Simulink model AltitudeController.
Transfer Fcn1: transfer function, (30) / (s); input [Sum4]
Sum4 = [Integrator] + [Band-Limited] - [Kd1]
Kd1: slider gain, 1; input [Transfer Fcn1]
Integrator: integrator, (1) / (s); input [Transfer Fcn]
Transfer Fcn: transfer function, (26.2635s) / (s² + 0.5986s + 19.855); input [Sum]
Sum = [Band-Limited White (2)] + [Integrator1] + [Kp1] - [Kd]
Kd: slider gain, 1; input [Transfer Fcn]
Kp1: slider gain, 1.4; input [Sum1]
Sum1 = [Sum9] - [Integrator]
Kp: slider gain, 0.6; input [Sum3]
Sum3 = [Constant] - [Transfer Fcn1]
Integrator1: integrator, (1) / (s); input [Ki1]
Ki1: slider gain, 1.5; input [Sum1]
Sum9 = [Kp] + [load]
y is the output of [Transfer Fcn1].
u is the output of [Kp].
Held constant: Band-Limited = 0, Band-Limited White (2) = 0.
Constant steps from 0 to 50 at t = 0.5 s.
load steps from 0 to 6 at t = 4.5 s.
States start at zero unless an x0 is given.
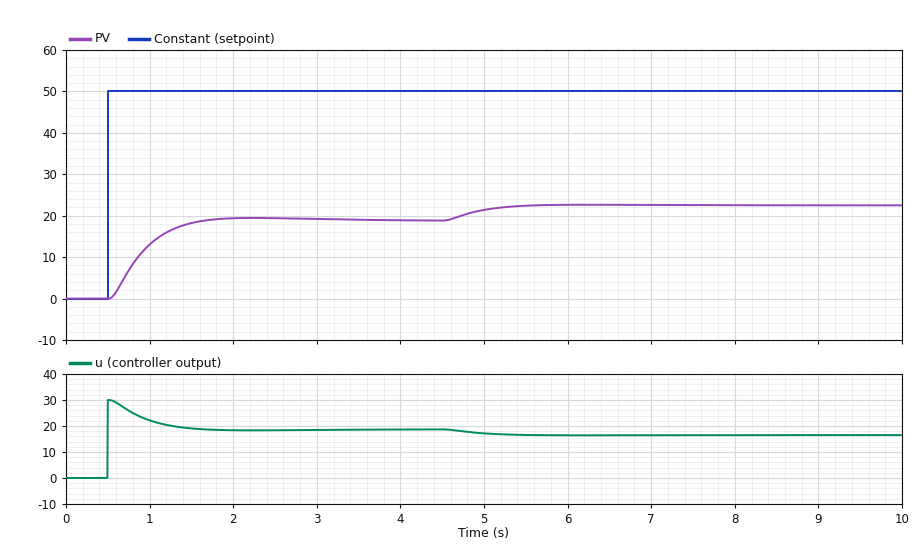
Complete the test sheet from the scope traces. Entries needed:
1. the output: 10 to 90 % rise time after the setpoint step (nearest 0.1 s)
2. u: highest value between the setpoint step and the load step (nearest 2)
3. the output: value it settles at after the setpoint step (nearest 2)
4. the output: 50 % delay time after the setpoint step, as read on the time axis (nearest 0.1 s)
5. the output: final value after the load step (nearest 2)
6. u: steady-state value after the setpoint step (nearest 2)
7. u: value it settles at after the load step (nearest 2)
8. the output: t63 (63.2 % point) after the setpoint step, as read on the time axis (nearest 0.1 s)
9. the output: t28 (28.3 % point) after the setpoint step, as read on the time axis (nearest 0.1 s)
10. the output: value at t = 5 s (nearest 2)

0.7 s
30
18
0.8 s
22
18
16
0.9 s
0.7 s
22
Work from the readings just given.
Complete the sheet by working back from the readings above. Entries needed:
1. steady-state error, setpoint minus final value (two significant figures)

32
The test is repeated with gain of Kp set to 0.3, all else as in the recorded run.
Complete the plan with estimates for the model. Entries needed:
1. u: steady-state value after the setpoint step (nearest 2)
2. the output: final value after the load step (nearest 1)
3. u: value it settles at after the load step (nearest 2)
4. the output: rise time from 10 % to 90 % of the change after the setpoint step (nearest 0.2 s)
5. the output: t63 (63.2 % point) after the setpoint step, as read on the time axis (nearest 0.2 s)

12
16
10
0.8 s
1.0 s
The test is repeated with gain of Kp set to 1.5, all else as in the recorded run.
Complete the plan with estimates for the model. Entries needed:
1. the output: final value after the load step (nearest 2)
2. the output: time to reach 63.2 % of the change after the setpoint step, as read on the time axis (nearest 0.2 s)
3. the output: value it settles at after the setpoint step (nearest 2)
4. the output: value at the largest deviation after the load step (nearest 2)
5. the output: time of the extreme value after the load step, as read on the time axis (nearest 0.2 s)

32
0.8 s
30
32
5.6 s
